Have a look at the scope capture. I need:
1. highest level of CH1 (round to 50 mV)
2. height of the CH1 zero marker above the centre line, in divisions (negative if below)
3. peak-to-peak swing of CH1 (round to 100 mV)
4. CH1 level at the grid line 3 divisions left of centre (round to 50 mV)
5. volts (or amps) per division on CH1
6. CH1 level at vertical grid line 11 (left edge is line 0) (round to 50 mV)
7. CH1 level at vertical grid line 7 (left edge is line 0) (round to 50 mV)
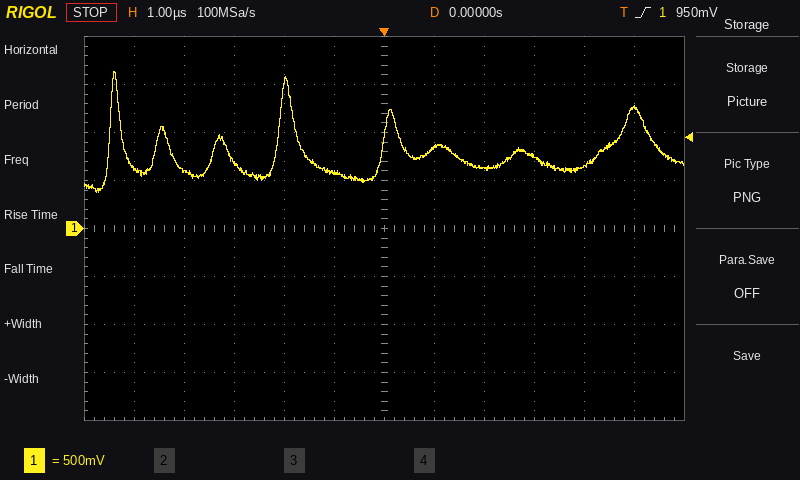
1.65 V
0.0 div
1.30 V
700 mV
500 mV
1.25 V
850 mV
